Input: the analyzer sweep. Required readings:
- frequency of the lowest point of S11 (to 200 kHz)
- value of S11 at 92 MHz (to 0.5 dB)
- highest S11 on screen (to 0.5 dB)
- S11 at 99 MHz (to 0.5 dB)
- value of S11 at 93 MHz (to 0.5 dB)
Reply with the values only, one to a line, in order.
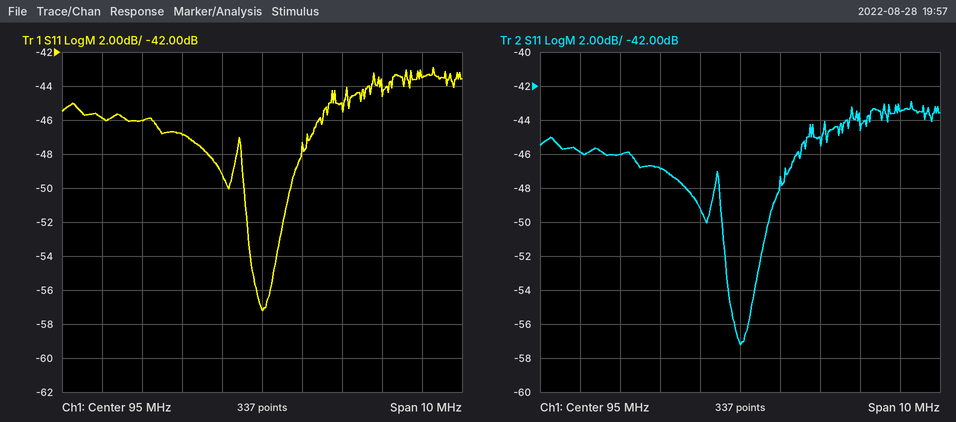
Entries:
95.0 MHz
-46.0 dB
-43.0 dB
-43.5 dB
-47.0 dB
